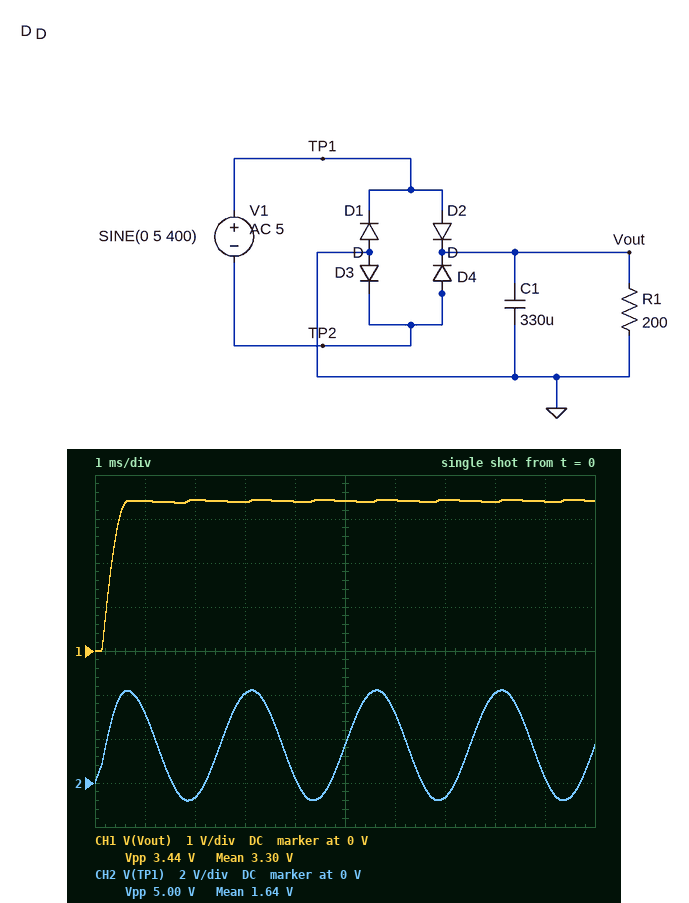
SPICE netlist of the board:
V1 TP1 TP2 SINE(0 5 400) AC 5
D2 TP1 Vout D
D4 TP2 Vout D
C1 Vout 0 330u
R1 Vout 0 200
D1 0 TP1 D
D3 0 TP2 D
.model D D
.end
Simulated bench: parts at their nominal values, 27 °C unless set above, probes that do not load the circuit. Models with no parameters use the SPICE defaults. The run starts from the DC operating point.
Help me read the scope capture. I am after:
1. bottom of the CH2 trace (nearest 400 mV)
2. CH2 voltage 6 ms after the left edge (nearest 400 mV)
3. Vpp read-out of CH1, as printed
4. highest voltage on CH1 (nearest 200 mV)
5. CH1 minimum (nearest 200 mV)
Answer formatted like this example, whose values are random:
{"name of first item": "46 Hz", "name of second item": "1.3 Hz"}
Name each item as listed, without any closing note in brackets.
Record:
{"bottom of the CH2 trace": "-800 mV", "CH2 voltage 6 ms after the left edge": "3.2 V", "Vpp read-out of CH1, as printed": "3.44 V", "highest voltage on CH1": "3.4 V", "CH1 minimum": "0 V"}
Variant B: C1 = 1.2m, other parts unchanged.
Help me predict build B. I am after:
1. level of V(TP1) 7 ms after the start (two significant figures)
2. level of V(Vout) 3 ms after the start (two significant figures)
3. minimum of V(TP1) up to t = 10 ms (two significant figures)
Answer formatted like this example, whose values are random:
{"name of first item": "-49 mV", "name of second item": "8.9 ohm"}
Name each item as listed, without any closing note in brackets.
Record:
{"level of V(TP1) 7 ms after the start": "-670 mV", "level of V(Vout) 3 ms after the start": "3.4 V", "minimum of V(TP1) up to t = 10 ms": "-820 mV"}
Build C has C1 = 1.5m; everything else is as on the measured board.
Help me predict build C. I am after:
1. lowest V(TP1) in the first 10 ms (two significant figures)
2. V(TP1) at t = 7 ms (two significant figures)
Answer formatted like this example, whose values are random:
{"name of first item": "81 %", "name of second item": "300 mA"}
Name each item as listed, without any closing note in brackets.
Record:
{"lowest V(TP1) in the first 10 ms": "-820 mV", "V(TP1) at t = 7 ms": "-670 mV"}
